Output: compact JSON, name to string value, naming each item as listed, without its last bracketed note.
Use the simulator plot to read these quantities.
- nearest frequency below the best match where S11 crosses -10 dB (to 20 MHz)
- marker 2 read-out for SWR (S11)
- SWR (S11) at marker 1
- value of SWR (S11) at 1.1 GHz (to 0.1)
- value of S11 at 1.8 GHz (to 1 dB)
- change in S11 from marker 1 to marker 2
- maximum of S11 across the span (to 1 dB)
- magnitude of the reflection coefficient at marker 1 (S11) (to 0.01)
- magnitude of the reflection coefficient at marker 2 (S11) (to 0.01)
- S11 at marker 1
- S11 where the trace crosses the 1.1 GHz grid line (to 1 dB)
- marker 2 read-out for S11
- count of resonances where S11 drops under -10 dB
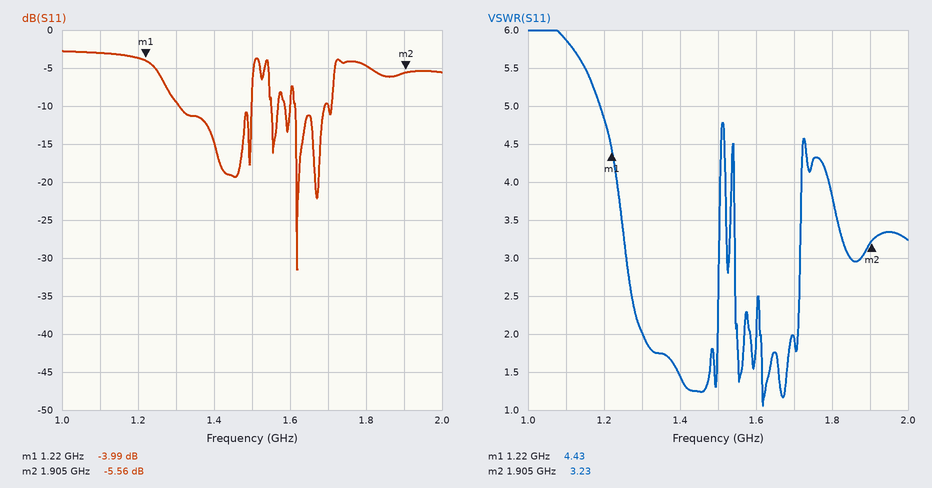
{"nearest frequency below the best match where S11 crosses -10 dB": "1.62 GHz", "marker 2 read-out for SWR": "3.23", "SWR (S11) at marker 1": "4.43", "value of SWR (S11) at 1.1 GHz": "5.9", "value of S11 at 1.8 GHz": "-5 dB", "change in S11 from marker 1 to marker 2": "-1.57 dB", "maximum of S11 across the span": "-3 dB", "magnitude of the reflection coefficient at marker 1 (S11)": "0.63", "magnitude of the reflection coefficient at marker 2 (S11)": "0.53", "S11 at marker 1": "-3.99 dB", "S11 where the trace crosses the 1.1 GHz grid line": "-3 dB", "marker 2 read-out for S11": "-5.56 dB", "count of resonances where S11 drops under -10 dB": "6"}
